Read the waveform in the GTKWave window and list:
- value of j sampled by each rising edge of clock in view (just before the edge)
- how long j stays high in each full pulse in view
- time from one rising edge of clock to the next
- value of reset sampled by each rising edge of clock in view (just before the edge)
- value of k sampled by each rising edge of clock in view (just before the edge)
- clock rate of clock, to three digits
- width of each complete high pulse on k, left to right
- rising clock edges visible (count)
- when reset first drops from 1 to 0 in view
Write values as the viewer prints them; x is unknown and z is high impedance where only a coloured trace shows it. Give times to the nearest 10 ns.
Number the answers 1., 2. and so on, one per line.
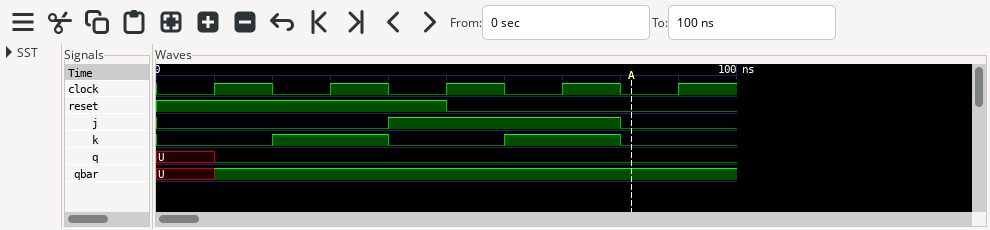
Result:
1. 0 0 1 1 0
2. 40 ns
3. 20 ns
4. 1 1 1 0 0
5. 0 1 0 1 0
6. 50.0 MHz
7. 20 ns, 20 ns
8. 5
9. 50 ns
